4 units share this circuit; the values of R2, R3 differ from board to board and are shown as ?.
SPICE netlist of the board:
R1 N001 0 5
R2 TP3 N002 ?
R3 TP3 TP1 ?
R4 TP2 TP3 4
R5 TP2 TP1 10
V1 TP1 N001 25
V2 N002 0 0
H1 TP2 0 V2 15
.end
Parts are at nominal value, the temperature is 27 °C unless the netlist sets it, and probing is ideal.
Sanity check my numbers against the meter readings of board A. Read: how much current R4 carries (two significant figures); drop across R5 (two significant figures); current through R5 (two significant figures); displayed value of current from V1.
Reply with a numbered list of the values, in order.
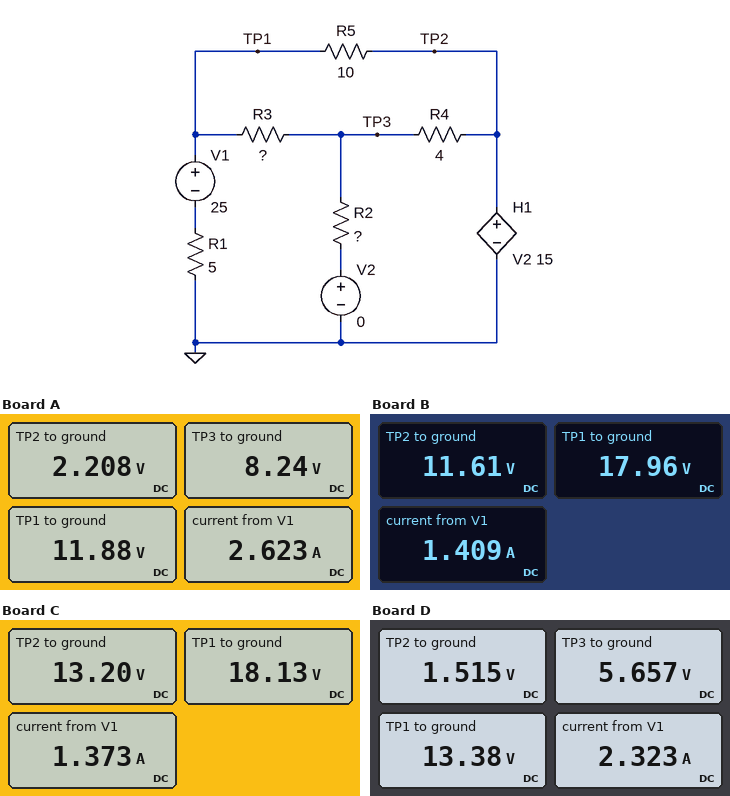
1. 1.5 A
2. 9.7 V
3. 970 mA
4. 2.623 A
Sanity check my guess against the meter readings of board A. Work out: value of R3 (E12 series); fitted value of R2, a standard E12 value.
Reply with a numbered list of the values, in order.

1. 2.2 Ω
2. 56 Ω
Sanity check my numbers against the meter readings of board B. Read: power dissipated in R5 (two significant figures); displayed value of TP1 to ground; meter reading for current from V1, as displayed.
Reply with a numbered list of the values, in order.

1. 4.0 W
2. 17.96 V
3. 1.409 A
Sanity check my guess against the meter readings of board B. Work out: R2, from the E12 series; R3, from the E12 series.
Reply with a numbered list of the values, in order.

1. 15 Ω
2. 8.2 Ω
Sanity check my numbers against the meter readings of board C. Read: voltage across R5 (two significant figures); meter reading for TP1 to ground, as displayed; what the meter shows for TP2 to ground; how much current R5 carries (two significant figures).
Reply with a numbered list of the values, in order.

1. 4.9 V
2. 18.13 V
3. 13.20 V
4. 490 mA
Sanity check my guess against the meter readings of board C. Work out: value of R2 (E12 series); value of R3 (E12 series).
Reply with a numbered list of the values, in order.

1. 15 Ω
2. 5.6 Ω
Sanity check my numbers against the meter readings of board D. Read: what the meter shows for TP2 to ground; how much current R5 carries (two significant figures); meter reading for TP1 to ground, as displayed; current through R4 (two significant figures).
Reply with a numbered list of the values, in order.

1. 1.515 V
2. 1.2 A
3. 13.38 V
4. 1.0 A
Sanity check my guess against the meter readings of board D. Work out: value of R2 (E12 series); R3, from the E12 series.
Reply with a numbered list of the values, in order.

1. 56 Ω
2. 6.8 Ω
